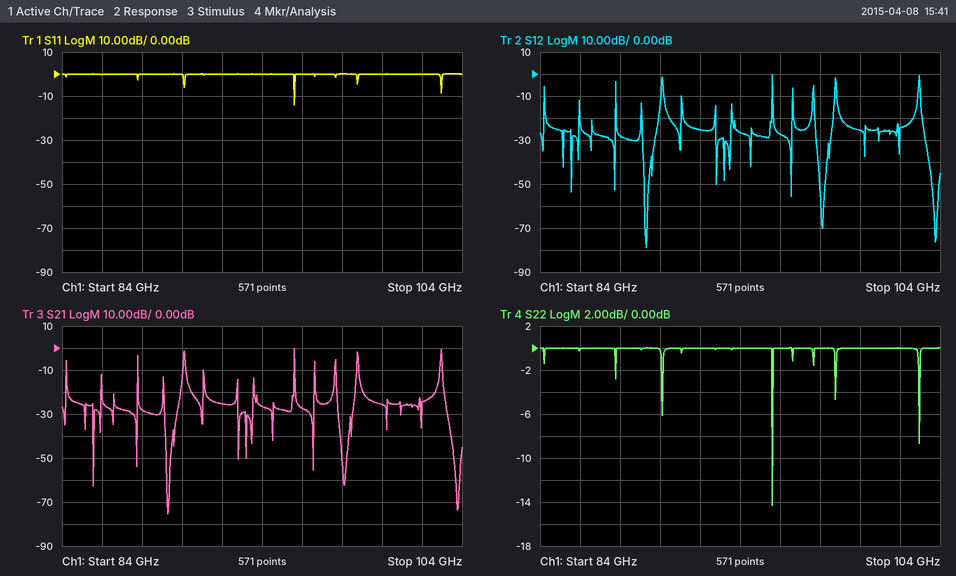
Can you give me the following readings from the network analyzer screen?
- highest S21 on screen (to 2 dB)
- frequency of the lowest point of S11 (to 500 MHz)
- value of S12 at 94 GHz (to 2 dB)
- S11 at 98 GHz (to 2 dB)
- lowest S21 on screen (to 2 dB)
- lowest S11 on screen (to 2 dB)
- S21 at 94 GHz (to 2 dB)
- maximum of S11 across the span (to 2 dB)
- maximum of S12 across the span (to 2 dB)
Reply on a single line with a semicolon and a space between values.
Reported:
0 dB; 95.5 GHz; -26 dB; 0 dB; -76 dB; -14 dB; -26 dB; 0 dB; 0 dB
